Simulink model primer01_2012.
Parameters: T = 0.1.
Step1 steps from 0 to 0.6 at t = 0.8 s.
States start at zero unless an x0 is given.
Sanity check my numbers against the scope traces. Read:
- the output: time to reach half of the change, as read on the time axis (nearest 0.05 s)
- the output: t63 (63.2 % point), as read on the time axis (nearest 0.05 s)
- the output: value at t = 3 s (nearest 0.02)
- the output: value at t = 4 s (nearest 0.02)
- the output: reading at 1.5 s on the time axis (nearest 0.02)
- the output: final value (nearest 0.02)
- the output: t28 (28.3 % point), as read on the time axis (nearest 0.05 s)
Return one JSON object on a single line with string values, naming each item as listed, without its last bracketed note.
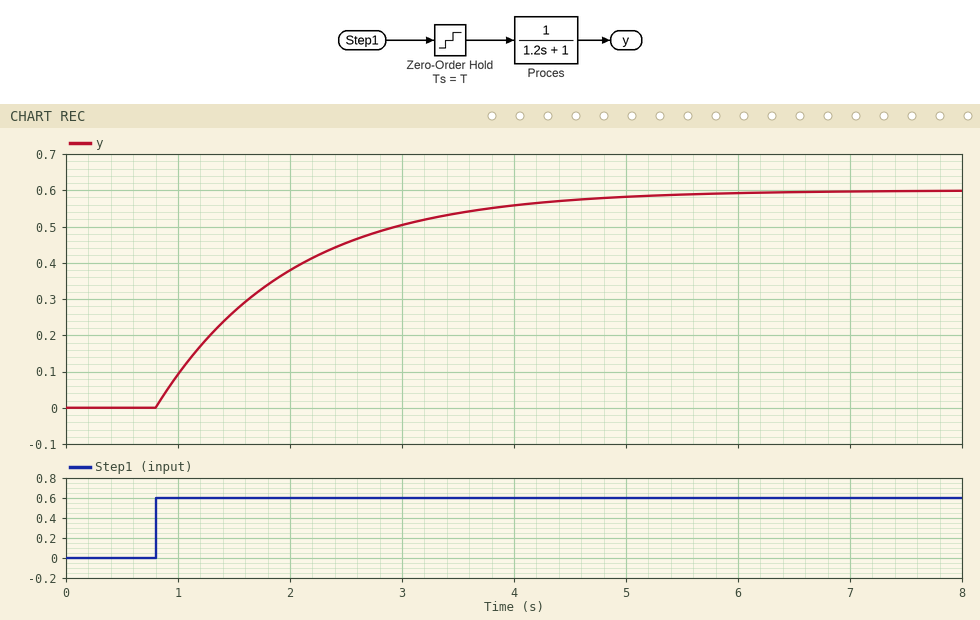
{"the output: time to reach half of the change, as read on the time axis": "1.65 s", "the output: t63 (63.2 % point), as read on the time axis": "2.00 s", "the output: value at t = 3 s": "0.50", "the output: value at t = 4 s": "0.56", "the output: reading at 1.5 s on the time axis": "0.26", "the output: final value": "0.60", "the output: t28 (28.3 % point), as read on the time axis": "1.20 s"}
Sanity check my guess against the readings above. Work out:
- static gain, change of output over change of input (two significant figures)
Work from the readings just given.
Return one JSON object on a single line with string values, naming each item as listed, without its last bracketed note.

{"static gain, change of output over change of input": "1.0"}
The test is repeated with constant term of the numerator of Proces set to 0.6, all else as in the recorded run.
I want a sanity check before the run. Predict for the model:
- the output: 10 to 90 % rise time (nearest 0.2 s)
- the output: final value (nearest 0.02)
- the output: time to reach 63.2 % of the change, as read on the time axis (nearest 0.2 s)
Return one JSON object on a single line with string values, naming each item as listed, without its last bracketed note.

{"the output: 10 to 90 % rise time": "2.6 s", "the output: final value": "0.36", "the output: time to reach 63.2 % of the change, as read on the time axis": "2.0 s"}
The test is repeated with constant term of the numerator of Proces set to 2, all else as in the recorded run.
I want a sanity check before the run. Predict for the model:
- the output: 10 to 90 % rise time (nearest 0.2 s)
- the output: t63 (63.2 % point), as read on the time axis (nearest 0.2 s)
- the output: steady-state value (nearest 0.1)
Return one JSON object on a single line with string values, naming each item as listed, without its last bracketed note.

{"the output: 10 to 90 % rise time": "2.6 s", "the output: t63 (63.2 % point), as read on the time axis": "2.0 s", "the output: steady-state value": "1.2"}
